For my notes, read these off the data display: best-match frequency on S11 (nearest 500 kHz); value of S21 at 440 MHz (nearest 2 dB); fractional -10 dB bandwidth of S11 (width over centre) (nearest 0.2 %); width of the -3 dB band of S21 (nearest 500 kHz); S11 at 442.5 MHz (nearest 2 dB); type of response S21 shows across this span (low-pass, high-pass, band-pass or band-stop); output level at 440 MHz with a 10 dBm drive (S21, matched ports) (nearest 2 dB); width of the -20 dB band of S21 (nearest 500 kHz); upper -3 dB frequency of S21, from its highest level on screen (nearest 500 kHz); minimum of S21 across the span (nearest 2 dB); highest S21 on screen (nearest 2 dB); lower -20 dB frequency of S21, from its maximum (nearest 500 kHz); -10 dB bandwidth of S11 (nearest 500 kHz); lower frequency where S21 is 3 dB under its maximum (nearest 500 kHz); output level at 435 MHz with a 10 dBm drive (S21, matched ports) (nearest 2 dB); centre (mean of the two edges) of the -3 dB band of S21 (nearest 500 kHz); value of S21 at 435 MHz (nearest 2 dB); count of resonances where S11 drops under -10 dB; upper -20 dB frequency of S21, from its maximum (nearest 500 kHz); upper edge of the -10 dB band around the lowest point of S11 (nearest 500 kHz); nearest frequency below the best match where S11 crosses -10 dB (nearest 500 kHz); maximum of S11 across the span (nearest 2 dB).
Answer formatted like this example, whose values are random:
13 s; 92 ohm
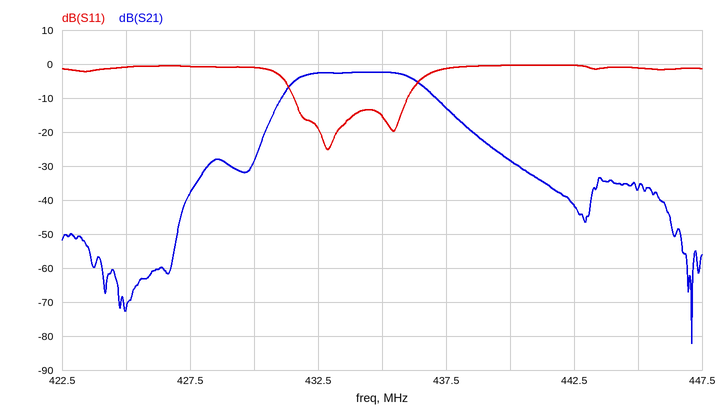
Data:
433.0 MHz; -28 dB; 1.0 %; 5.0 MHz; 0 dB; band-pass; -18 dBm; 8.5 MHz; 436.5 MHz; -82 dB; -2 dB; 430.5 MHz; 4.5 MHz; 431.5 MHz; 8 dBm; 434.0 MHz; -2 dB; 2; 439.0 MHz; 436.0 MHz; 431.5 MHz; 0 dB
